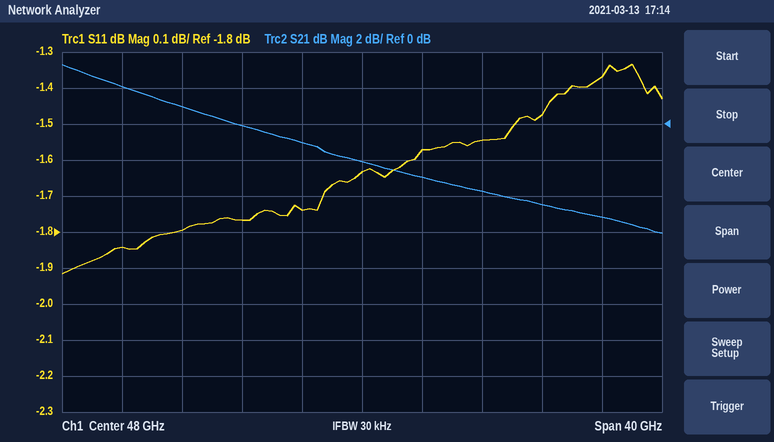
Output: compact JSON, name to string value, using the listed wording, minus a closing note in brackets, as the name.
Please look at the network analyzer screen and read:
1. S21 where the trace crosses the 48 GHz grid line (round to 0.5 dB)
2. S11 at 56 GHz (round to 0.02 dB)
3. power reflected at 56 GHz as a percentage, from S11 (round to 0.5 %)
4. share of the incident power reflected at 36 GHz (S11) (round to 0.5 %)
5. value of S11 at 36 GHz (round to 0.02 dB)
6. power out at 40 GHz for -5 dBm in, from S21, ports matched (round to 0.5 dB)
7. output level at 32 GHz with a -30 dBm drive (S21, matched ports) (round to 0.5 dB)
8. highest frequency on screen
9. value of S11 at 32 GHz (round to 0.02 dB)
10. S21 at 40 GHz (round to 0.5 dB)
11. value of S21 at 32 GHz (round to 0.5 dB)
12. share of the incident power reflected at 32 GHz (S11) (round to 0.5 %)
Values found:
{"S21 where the trace crosses the 48 GHz grid line": "-2.0 dB", "S11 at 56 GHz": "-1.54 dB", "power reflected at 56 GHz as a percentage, from S11": "70.0 %", "share of the incident power reflected at 36 GHz (S11)": "66.0 %", "value of S11 at 36 GHz": "-1.80 dB", "power out at 40 GHz for -5 dBm in, from S21, ports matched": "-5.0 dBm", "output level at 32 GHz with a -30 dBm drive (S21, matched ports)": "-28.0 dBm", "highest frequency on screen": "68 GHz", "value of S11 at 32 GHz": "-1.84 dB", "S21 at 40 GHz": "0.0 dB", "value of S21 at 32 GHz": "2.0 dB", "share of the incident power reflected at 32 GHz (S11)": "65.5 %"}
